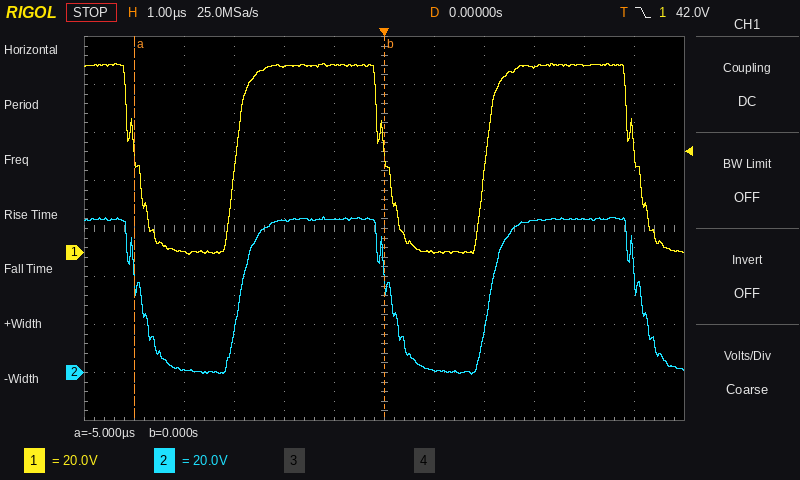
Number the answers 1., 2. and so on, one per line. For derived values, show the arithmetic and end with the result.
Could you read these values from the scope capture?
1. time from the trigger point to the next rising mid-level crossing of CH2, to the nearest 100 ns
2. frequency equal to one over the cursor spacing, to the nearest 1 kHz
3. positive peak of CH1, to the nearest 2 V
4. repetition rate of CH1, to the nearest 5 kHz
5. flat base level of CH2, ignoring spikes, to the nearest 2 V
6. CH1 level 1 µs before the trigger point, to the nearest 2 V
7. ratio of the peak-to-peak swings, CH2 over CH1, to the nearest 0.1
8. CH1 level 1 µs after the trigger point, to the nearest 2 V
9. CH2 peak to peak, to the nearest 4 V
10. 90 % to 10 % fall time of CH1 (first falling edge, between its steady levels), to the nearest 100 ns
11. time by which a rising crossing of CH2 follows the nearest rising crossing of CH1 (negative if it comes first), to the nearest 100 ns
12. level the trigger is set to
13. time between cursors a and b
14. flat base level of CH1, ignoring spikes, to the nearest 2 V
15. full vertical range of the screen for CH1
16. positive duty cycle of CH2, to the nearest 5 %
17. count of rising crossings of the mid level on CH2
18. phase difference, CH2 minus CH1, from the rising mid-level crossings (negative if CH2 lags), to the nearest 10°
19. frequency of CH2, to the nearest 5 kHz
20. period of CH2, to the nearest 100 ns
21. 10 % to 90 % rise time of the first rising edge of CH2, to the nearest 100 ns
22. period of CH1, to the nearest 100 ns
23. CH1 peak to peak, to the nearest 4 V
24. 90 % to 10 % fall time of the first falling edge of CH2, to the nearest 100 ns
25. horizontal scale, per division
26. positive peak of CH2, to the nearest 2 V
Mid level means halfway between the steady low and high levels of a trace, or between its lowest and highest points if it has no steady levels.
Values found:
1. 2.1 µs
2. 1 / 5.0 µs ≈ 200 kHz
3. 78 V
4. 1 / 5.0 µs ≈ 200 kHz
5. 0 V
6. 78 V
7. 64 V / 80 V ≈ 0.8
8. 0 V
9. 64 V
10. 600 ns
11. +100 ns
12. 42.0 V
13. 0 s − (-5 µs) = 5.0 µs
14. 0 V
15. 160 V
16. 60 %
17. 2
18. −360° × (+100 ns) / 5.0 µs ≈ -7.20°, so -10° to the nearest 10°
19. 1 / 5.0 µs ≈ 200 kHz
20. 5.0 µs
21. 600 ns
22. 5.0 µs
23. 80 V
24. 700 ns
25. 1 µs
26. 64 V
